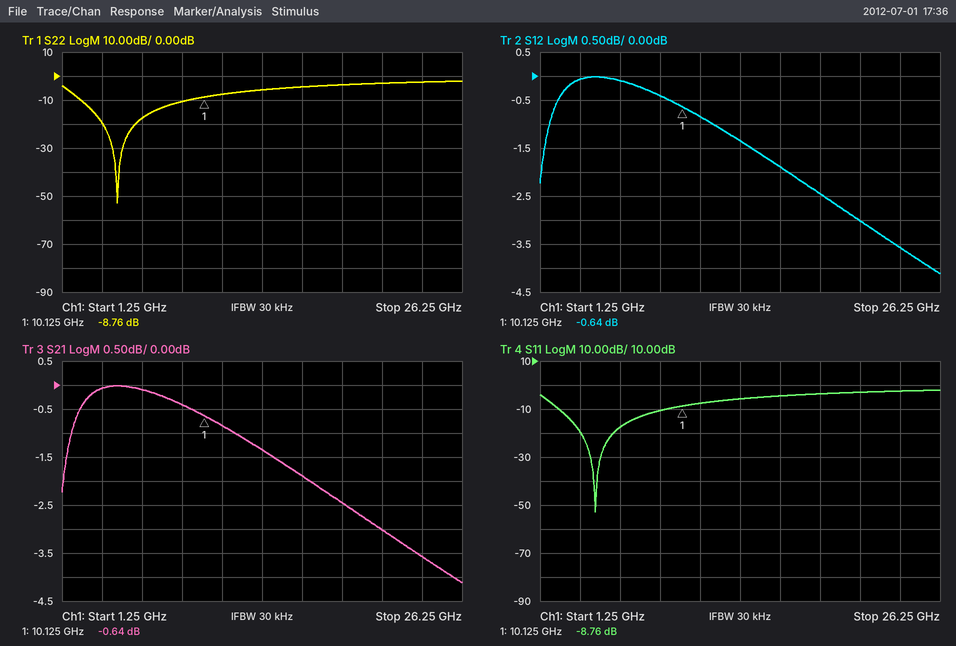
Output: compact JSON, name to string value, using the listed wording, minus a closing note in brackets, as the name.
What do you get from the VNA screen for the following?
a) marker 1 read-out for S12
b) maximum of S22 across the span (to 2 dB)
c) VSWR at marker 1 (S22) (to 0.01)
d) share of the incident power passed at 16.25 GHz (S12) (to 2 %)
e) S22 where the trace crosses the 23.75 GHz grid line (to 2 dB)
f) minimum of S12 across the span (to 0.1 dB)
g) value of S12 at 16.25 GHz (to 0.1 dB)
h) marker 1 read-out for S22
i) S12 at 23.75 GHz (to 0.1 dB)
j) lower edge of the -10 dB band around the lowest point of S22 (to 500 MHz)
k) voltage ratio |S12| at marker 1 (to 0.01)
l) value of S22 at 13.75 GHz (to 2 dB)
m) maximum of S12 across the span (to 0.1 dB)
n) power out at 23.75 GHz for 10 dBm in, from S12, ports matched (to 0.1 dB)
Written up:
{"marker 1 read-out for S12": "-0.64 dB", "maximum of S22 across the span": "-2 dB", "VSWR at marker 1 (S22)": "2.15", "share of the incident power passed at 16.25 GHz (S12)": "64 %", "S22 where the trace crosses the 23.75 GHz grid line": "-2 dB", "minimum of S12 across the span": "-4.1 dB", "value of S12 at 16.25 GHz": "-1.9 dB", "marker 1 read-out for S22": "-8.76 dB", "S12 at 23.75 GHz": "-3.6 dB", "lower edge of the -10 dB band around the lowest point of S22": "2.5 GHz", "voltage ratio |S12| at marker 1": "0.93", "value of S22 at 13.75 GHz": "-6 dB", "maximum of S12 across the span": "0.0 dB", "power out at 23.75 GHz for 10 dBm in, from S12, ports matched": "6.4 dBm"}
